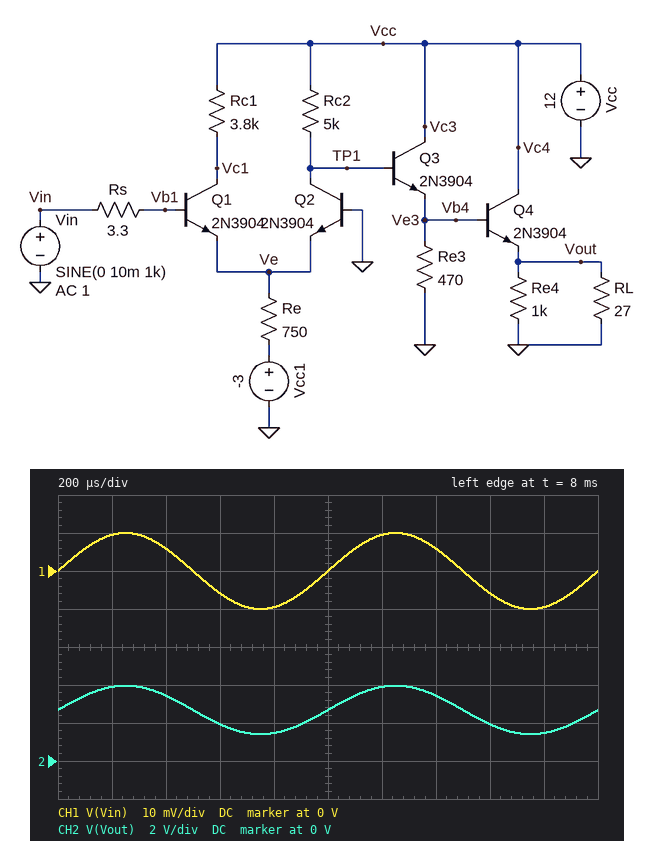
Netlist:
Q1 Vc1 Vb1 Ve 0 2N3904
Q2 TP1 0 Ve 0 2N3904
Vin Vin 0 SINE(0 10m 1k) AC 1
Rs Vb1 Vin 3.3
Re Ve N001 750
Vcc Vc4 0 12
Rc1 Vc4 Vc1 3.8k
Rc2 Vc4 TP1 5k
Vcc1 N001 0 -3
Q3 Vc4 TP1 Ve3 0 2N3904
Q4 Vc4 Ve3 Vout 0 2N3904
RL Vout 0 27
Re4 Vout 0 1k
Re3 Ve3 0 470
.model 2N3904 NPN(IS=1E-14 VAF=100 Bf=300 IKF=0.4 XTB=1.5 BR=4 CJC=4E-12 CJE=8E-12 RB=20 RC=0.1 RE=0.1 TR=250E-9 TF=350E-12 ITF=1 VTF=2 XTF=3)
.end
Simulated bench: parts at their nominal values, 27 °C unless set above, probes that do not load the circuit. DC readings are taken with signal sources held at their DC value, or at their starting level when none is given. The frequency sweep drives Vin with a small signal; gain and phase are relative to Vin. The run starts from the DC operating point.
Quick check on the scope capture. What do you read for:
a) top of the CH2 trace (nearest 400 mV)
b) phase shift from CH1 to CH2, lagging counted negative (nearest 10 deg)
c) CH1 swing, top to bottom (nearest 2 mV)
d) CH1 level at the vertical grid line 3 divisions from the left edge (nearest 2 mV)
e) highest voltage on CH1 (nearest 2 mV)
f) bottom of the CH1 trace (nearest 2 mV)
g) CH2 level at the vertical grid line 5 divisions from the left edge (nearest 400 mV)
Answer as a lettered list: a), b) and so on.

a) 4.0 V
b) 0 deg
c) 20 mV
d) -6 mV
e) 10 mV
f) -10 mV
g) 2.8 V
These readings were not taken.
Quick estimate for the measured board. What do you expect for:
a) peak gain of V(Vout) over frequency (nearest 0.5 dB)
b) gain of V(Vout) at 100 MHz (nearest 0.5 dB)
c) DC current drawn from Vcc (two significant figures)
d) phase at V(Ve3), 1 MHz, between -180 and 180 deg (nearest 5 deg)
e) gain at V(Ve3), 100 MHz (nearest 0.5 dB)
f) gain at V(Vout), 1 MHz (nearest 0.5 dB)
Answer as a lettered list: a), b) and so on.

a) 42.0 dB
b) 10.0 dB
c) 110 mA
d) -10 deg
e) 10.5 dB
f) 42.0 dB
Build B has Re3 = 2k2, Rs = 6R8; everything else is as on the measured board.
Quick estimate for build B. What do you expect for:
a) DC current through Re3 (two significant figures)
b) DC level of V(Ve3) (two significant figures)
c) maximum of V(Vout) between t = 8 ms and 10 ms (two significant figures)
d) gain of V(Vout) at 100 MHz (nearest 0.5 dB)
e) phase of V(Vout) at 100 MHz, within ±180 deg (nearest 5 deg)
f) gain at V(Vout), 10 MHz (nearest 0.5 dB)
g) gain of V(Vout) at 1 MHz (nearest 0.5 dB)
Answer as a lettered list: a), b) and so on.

a) 1.6 mA
b) 3.6 V
c) 4.1 V
d) 8.5 dB
e) -140 deg
f) 35.5 dB
g) 42.5 dB
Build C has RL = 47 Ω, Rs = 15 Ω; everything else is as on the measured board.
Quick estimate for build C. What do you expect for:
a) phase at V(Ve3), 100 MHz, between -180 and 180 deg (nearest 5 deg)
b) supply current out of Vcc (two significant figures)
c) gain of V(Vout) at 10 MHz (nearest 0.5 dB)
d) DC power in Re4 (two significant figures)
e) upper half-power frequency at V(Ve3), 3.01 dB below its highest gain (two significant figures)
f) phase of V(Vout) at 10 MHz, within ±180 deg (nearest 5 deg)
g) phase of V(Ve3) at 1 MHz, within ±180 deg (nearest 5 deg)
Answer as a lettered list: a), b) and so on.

a) -120 deg
b) 71 mA
c) 34.5 dB
d) 7.3 mW
e) 4.8 MHz
f) -80 deg
g) -15 deg
